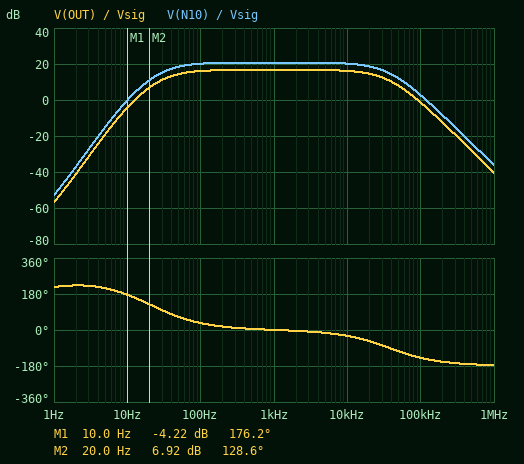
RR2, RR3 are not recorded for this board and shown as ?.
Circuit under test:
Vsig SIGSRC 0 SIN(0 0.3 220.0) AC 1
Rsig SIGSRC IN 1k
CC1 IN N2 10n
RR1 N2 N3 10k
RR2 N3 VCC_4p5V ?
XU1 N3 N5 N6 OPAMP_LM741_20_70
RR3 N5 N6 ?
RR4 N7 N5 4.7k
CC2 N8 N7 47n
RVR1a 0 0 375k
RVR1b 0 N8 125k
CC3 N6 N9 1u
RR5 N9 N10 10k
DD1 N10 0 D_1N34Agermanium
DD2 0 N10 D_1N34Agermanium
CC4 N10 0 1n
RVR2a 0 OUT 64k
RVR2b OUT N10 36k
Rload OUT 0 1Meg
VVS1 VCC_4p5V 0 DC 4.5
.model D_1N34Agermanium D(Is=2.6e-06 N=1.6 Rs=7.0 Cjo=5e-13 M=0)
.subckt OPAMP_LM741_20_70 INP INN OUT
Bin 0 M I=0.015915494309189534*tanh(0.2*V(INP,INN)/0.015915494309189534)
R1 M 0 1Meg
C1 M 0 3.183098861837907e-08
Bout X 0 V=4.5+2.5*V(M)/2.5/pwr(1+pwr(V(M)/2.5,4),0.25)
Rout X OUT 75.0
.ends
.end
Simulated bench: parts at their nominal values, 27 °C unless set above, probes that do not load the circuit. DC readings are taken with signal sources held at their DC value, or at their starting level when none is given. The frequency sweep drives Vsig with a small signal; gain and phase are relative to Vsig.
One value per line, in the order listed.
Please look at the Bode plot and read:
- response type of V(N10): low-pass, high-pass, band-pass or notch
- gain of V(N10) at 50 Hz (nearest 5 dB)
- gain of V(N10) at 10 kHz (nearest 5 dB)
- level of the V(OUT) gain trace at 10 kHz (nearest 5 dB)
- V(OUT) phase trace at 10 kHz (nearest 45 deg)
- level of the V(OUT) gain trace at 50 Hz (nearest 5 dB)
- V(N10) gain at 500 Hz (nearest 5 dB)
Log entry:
band-pass
20 dB
20 dB
15 dB
-45 deg
15 dB
20 dB
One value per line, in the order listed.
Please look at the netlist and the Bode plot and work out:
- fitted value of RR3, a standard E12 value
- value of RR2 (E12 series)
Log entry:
3.3 MΩ
560 kΩ
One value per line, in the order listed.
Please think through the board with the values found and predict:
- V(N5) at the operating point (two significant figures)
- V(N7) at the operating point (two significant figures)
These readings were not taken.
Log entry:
4.5 V
4.5 V
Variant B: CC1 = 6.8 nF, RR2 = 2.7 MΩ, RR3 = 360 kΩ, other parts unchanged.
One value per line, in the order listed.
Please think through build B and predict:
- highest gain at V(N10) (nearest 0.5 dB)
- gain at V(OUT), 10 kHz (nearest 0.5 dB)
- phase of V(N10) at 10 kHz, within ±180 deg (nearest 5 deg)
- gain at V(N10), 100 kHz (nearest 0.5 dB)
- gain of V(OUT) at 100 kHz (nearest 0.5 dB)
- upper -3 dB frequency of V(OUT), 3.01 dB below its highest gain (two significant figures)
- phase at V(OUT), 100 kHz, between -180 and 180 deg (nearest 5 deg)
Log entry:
4.0 dB
-0.5 dB
-15 deg
-5.5 dB
-9.5 dB
37 kHz
-90 deg
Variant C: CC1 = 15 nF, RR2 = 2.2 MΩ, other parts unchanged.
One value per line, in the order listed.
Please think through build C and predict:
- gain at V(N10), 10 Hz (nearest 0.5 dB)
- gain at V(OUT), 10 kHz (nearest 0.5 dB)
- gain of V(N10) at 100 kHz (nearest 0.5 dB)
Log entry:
8.5 dB
16.5 dB
3.0 dB
